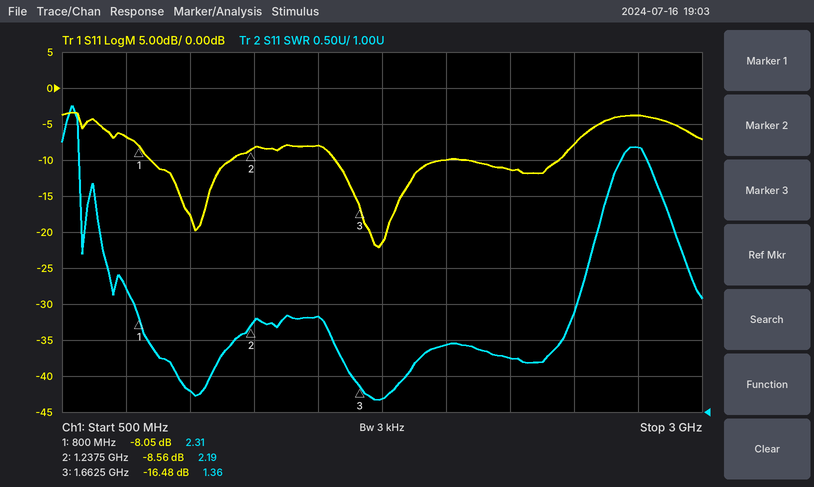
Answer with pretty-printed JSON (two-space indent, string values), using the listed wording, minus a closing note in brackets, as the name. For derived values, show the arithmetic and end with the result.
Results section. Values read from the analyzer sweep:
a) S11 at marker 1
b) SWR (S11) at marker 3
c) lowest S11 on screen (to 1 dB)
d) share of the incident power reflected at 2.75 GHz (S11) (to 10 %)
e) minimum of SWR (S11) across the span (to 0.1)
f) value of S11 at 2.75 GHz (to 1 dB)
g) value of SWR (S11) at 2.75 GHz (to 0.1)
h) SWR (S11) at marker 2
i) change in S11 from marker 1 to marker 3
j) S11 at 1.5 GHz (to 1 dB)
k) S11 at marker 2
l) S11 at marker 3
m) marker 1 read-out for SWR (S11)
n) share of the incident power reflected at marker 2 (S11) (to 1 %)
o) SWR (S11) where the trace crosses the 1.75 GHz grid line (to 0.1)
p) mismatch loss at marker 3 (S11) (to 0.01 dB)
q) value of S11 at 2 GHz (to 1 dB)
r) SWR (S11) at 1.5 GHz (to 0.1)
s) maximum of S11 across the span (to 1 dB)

{
  "S11 at marker 1": "-8.05 dB",
  "SWR (S11) at marker 3": "1.36",
  "lowest S11 on screen": "-22 dB",
  "share of the incident power reflected at 2.75 GHz (S11)": "10^(-4/10) ≈ 40 %",
  "minimum of SWR (S11) across the span": "1.2",
  "value of S11 at 2.75 GHz": "-4 dB",
  "value of SWR (S11) at 2.75 GHz": "4.7",
  "SWR (S11) at marker 2": "2.19",
  "change in S11 from marker 1 to marker 3": "-16.48 − (-8.05) = -8.43 dB",
  "S11 at 1.5 GHz": "-8 dB",
  "S11 at marker 2": "-8.56 dB",
  "S11 at marker 3": "-16.48 dB",
  "marker 1 read-out for SWR": "2.31",
  "share of the incident power reflected at marker 2 (S11)": "10^(-8.56/10) ≈ 14 %",
  "SWR (S11) where the trace crosses the 1.75 GHz grid line": "1.2",
  "mismatch loss at marker 3 (S11)": "−10 log10(1 − 10^(-16.48/10)) ≈ 0.10 dB",
  "value of S11 at 2 GHz": "-10 dB",
  "SWR (S11) at 1.5 GHz": "2.3",
  "maximum of S11 across the span": "-3 dB"
}
